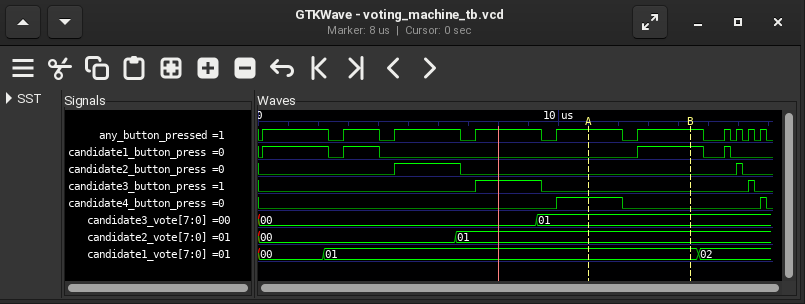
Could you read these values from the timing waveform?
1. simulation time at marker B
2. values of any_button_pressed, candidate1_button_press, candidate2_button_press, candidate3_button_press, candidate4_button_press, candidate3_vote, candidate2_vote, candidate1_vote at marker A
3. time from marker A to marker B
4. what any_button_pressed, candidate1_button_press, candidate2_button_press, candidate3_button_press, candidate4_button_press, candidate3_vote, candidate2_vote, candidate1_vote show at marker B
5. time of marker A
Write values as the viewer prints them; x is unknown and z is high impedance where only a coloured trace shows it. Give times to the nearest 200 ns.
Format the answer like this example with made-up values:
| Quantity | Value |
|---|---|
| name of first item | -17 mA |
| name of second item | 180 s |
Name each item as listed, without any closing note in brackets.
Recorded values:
| Quantity | Value |
|---|---|
| simulation time at marker B | 14400 ns |
| values of any_button_pressed, candidate1_button_press, candidate2_button_press, candidate3_button_press, candidate4_button_press, candidate3_vote, candidate2_vote, candidate1_vote at marker A | any_button_pressed=1, candidate1_button_press=0, candidate2_button_press=0, candidate3_button_press=0, candidate4_button_press=1, candidate3_vote=01, candidate2_vote=01, candidate1_vote=01 |
| time from marker A to marker B | 3400 ns |
| what any_button_pressed, candidate1_button_press, candidate2_button_press, candidate3_button_press, candidate4_button_press, candidate3_vote, candidate2_vote, candidate1_vote show at marker B | any_button_pressed=1, candidate1_button_press=1, candidate2_button_press=0, candidate3_button_press=0, candidate4_button_press=0, candidate3_vote=01, candidate2_vote=01, candidate1_vote=01 |
| time of marker A | 11000 ns |
